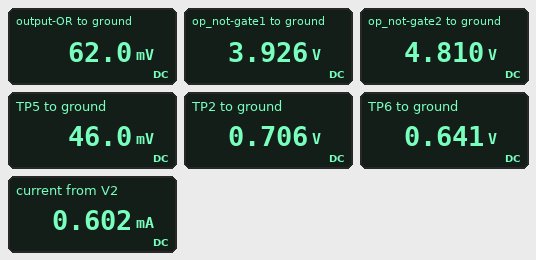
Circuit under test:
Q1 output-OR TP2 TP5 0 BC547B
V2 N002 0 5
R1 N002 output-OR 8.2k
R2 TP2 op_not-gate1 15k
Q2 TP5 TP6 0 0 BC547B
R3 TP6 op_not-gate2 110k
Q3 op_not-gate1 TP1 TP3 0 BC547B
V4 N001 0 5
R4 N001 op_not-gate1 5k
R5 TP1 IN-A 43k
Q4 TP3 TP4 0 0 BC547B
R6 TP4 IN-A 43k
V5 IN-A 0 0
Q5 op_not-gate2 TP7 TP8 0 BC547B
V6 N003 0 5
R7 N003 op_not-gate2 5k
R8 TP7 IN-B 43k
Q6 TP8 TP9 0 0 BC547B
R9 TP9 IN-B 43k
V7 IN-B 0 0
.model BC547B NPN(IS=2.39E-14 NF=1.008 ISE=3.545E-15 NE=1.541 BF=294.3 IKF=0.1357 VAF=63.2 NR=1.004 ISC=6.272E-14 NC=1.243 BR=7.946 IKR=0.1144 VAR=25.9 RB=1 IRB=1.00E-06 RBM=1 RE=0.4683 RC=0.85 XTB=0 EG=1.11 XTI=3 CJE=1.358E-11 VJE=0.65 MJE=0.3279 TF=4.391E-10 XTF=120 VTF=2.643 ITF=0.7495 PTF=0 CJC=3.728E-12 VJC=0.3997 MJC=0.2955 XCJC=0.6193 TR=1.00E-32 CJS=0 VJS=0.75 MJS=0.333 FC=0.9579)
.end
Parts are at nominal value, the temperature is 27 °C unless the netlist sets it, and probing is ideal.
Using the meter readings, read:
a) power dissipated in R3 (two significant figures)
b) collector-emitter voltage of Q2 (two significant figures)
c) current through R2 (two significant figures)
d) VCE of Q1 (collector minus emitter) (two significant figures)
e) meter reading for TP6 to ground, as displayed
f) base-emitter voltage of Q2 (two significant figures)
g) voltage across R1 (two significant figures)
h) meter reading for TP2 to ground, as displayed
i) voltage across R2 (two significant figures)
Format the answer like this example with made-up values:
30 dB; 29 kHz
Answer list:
160 µW; 46 mV; 210 µA; 16 mV; 0.641 V; 640 mV; 4.9 V; 0.706 V; 3.2 V
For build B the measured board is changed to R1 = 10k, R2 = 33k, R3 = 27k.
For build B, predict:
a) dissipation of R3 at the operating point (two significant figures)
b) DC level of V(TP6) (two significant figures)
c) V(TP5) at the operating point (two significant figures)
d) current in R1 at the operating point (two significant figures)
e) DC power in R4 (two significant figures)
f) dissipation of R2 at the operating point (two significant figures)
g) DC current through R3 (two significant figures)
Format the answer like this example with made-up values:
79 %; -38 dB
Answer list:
500 µW; 650 mV; 20 mV; 500 µA; 65 µW; 430 µW; 140 µA
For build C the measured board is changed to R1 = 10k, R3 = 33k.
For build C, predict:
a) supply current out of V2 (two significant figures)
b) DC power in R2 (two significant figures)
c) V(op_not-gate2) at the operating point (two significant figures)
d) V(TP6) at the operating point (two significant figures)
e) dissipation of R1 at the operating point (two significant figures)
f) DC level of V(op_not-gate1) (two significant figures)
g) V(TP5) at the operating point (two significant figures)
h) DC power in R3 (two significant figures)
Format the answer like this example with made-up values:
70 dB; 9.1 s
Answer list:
500 µA; 700 µW; 4.4 V; 650 mV; 2.5 mW; 3.9 V; 24 mV; 430 µW
